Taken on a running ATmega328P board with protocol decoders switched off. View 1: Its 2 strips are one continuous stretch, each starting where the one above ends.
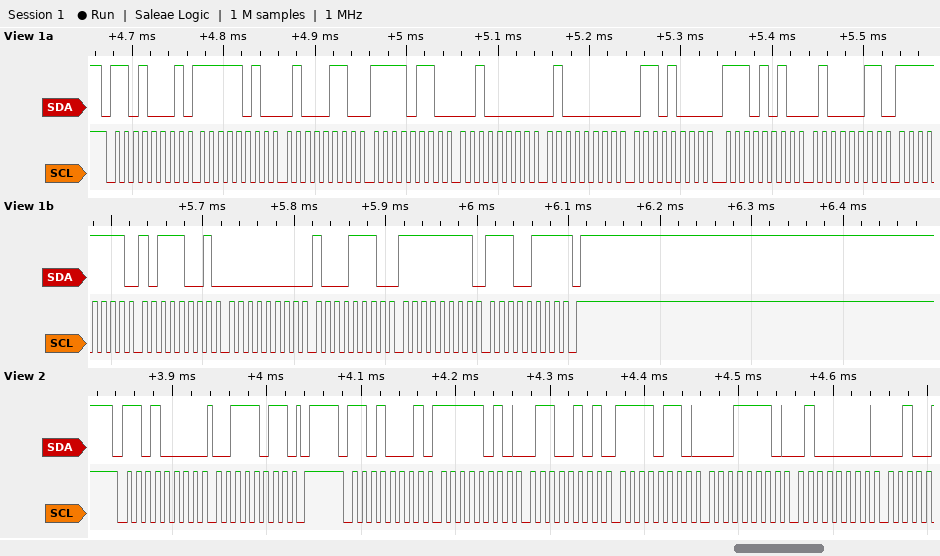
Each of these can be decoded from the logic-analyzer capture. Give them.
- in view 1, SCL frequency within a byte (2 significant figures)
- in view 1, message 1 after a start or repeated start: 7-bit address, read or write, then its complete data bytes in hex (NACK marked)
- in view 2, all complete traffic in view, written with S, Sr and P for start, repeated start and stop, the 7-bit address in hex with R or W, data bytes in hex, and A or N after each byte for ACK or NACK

100 kHz
0x68 read: FA 46 F6 20 40 68 EA 43 FF B9 00 8E FF E7 NACK
S 68W A 3B A P S 68R A FA A 65 A F6 A 1E A 40 A
